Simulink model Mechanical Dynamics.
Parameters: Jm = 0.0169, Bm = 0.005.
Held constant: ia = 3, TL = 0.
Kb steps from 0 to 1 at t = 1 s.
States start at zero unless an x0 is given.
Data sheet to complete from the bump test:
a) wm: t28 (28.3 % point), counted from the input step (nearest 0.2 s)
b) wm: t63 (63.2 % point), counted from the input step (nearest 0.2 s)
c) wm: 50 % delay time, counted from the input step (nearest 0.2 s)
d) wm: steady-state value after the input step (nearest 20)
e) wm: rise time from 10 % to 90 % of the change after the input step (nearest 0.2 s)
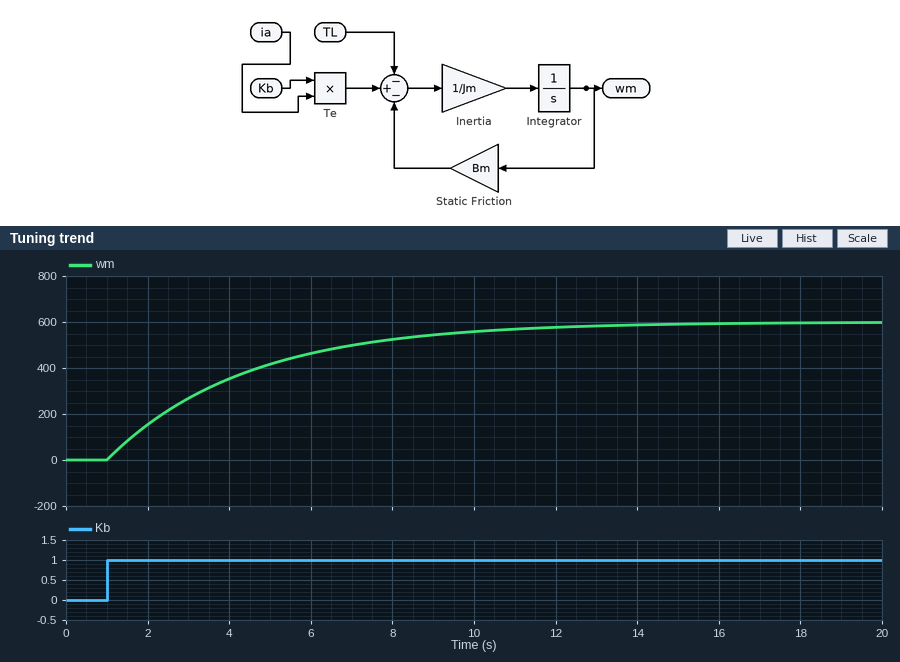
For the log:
1.2 s
3.4 s
2.4 s
600
7.4 s
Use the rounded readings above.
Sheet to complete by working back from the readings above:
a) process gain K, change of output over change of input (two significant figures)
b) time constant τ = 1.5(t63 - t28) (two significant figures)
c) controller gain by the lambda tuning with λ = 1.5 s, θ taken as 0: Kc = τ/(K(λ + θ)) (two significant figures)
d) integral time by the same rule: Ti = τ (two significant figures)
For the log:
600
3.3 s
0.0037
3.3 s
